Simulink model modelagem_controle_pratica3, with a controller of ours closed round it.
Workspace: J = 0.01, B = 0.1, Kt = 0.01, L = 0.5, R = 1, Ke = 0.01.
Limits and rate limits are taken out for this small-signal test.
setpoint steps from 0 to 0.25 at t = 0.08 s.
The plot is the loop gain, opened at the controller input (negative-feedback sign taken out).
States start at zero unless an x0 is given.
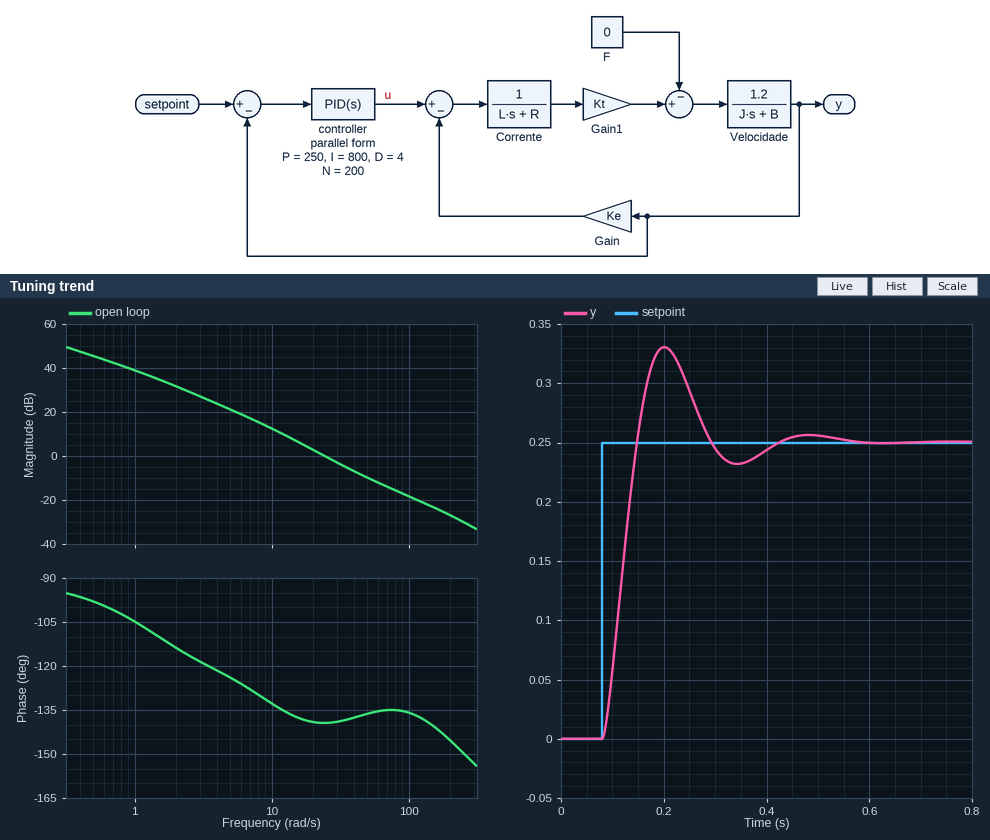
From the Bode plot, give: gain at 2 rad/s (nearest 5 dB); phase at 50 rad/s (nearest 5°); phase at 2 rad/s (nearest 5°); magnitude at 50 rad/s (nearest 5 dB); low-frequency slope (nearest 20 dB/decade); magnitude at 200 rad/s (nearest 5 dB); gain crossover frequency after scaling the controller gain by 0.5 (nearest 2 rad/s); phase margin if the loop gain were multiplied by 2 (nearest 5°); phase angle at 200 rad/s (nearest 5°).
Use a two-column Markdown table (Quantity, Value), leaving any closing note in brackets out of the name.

| Quantity | Value |
|---|---|
| gain at 2 rad/s | 30 dB |
| phase at 50 rad/s | -135° |
| phase at 2 rad/s | -115° |
| magnitude at 50 rad/s | -10 dB |
| low-frequency slope | -20 dB/decade |
| magnitude at 200 rad/s | -25 dB |
| gain crossover frequency after scaling the controller gain by 0.5 | 16 rad/s |
| phase margin if the loop gain were multiplied by 2 | 40° |
| phase angle at 200 rad/s | -145° |
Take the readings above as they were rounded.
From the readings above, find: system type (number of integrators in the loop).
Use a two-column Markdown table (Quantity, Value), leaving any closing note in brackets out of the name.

| Quantity | Value |
|---|---|
| system type | 1 |
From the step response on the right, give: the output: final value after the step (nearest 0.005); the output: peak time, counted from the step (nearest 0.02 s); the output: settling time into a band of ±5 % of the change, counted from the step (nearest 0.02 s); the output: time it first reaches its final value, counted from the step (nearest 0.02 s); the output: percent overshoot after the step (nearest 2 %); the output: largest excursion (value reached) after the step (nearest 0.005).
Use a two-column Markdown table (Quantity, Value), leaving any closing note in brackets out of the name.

| Quantity | Value |
|---|---|
| the output: final value after the step | 0.250 |
| the output: peak time, counted from the step | 0.12 s |
| the output: settling time into a band of ±5 % of the change, counted from the step | 0.30 s |
| the output: time it first reaches its final value, counted from the step | 0.06 s |
| the output: percent overshoot after the step | 32 % |
| the output: largest excursion (value reached) after the step | 0.330 |
